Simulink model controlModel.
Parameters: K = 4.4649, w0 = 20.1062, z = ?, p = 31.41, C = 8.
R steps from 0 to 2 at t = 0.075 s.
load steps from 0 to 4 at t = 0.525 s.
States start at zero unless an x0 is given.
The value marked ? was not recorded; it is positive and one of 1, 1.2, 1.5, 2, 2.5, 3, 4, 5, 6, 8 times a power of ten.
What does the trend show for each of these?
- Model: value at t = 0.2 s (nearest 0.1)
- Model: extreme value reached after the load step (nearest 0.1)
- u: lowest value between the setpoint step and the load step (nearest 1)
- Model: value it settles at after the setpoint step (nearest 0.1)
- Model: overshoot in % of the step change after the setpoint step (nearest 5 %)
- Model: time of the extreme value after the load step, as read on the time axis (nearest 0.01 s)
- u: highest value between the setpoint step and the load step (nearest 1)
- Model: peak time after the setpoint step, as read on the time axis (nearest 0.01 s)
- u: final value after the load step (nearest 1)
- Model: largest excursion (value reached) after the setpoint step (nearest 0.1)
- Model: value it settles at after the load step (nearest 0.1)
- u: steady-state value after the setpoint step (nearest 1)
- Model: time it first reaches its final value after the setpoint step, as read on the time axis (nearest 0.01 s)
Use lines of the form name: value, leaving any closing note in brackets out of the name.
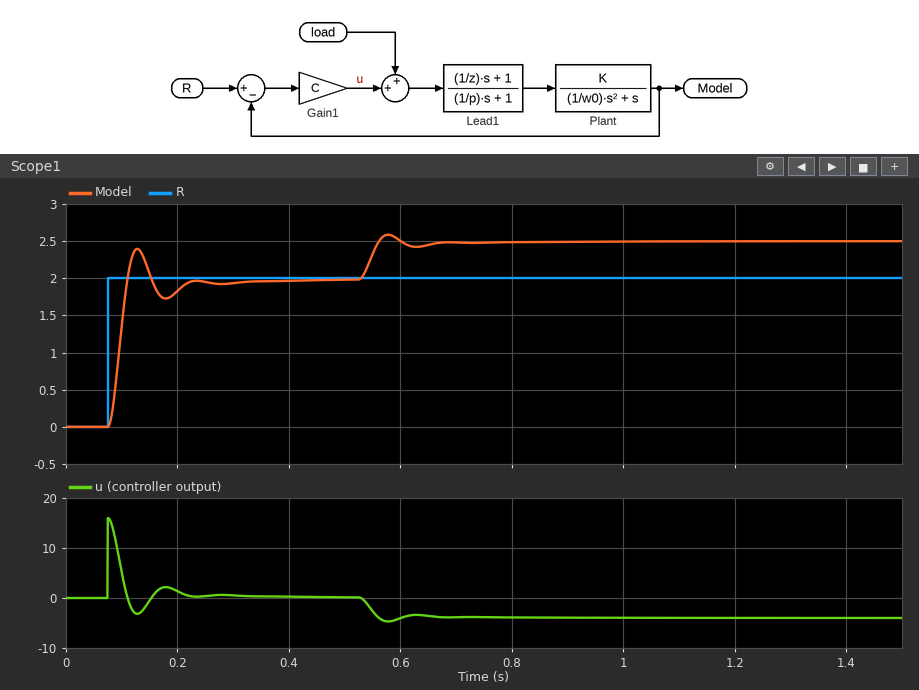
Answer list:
Model: value at t = 0.2 s: 1.8
Model: extreme value reached after the load step: 2.6
u: lowest value between the setpoint step and the load step: -3
Model: value it settles at after the setpoint step: 2.0
Model: overshoot in % of the step change after the setpoint step: 20 %
Model: time of the extreme value after the load step, as read on the time axis: 0.58 s
u: highest value between the setpoint step and the load step: 16
Model: peak time after the setpoint step, as read on the time axis: 0.13 s
u: final value after the load step: -4
Model: largest excursion (value reached) after the setpoint step: 2.4
Model: value it settles at after the load step: 2.5
u: steady-state value after the setpoint step: 0
Model: time it first reaches its final value after the setpoint step, as read on the time axis: 0.11 s
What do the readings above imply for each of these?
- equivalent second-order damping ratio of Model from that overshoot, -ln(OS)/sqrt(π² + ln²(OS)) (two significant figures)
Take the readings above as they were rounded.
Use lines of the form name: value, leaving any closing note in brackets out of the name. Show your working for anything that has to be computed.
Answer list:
equivalent second-order damping ratio of Model from that overshoot, -ln(OS)/sqrt(π² + ln²(OS)): ln(0.2) = -1.609; 1.609 / sqrt(9.870 + 2.590) = 0.46
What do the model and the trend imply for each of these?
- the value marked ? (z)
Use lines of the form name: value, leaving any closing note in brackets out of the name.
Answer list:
the value marked ?: 6
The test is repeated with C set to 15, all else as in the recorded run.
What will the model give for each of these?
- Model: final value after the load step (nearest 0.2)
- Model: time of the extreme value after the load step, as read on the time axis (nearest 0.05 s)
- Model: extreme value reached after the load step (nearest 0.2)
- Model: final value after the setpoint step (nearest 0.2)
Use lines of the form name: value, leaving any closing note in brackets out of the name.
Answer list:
Model: final value after the load step: 2.2
Model: time of the extreme value after the load step, as read on the time axis: 0.55 s
Model: extreme value reached after the load step: 2.4
Model: final value after the setpoint step: 2.0
